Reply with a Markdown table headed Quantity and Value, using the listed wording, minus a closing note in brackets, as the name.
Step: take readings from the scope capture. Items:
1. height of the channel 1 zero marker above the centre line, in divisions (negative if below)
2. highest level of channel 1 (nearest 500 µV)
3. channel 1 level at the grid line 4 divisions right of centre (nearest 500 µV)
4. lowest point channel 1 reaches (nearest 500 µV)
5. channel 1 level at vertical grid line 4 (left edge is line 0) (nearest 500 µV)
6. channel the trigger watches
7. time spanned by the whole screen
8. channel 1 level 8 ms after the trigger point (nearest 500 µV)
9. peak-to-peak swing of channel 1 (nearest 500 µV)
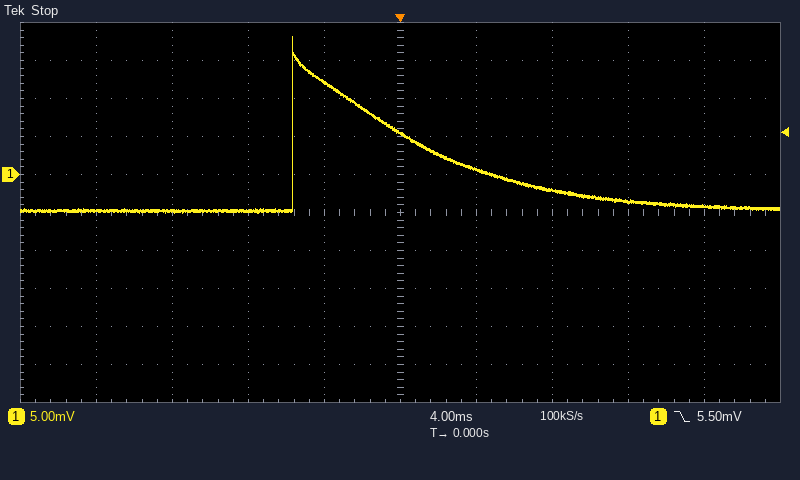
| Quantity | Value |
|---|---|
| height of the channel 1 zero marker above the centre line, in divisions | +1.0 div |
| highest level of channel 1 | 18.0 mV |
| channel 1 level at the grid line 4 divisions right of centre | -4.0 mV |
| lowest point channel 1 reaches | -5.0 mV |
| channel 1 level at vertical grid line 4 (left edge is line 0) | 12.0 mV |
| channel the trigger watches | channel 1 |
| time spanned by the whole screen | 40 ms |
| channel 1 level 8 ms after the trigger point | -2.0 mV |
| peak-to-peak swing of channel 1 | 23.0 mV |
